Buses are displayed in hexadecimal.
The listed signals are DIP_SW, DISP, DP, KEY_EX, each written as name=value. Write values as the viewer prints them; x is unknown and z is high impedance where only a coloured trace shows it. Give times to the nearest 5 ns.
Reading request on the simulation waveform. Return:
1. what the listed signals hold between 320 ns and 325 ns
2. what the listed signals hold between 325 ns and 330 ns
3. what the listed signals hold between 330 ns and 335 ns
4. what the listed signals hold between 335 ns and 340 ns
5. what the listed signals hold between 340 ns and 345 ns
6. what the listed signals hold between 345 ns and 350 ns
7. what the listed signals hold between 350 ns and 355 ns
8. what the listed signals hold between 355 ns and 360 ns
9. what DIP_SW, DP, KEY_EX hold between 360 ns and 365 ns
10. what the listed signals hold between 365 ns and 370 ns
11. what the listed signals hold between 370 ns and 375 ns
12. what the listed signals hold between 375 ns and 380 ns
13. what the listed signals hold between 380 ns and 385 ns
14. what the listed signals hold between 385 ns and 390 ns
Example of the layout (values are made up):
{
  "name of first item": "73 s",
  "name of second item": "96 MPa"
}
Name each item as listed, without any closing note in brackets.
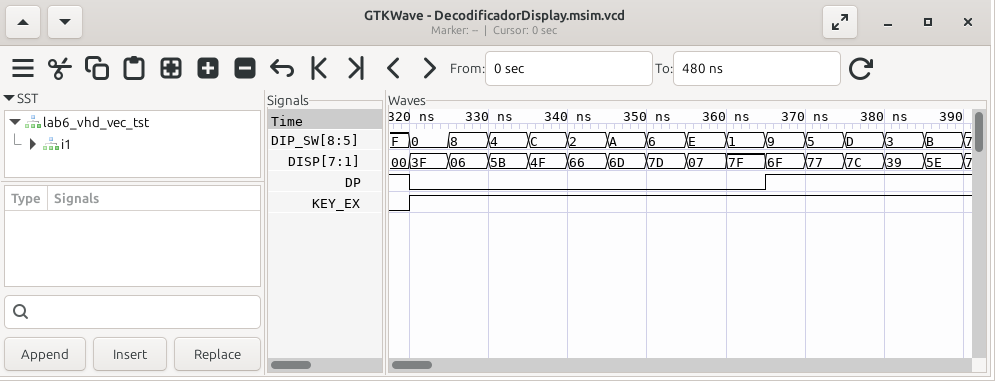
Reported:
{
  "what the listed signals hold between 320 ns and 325 ns": "DIP_SW=0, DISP=3F, DP=0, KEY_EX=1",
  "what the listed signals hold between 325 ns and 330 ns": "DIP_SW=8, DISP=06, DP=0, KEY_EX=1",
  "what the listed signals hold between 330 ns and 335 ns": "DIP_SW=4, DISP=5B, DP=0, KEY_EX=1",
  "what the listed signals hold between 335 ns and 340 ns": "DIP_SW=C, DISP=4F, DP=0, KEY_EX=1",
  "what the listed signals hold between 340 ns and 345 ns": "DIP_SW=2, DISP=66, DP=0, KEY_EX=1",
  "what the listed signals hold between 345 ns and 350 ns": "DIP_SW=A, DISP=6D, DP=0, KEY_EX=1",
  "what the listed signals hold between 350 ns and 355 ns": "DIP_SW=6, DISP=7D, DP=0, KEY_EX=1",
  "what the listed signals hold between 355 ns and 360 ns": "DIP_SW=E, DISP=07, DP=0, KEY_EX=1",
  "what DIP_SW, DP, KEY_EX hold between 360 ns and 365 ns": "DIP_SW=1, DP=0, KEY_EX=1",
  "what the listed signals hold between 365 ns and 370 ns": "DIP_SW=9, DISP=6F, DP=1, KEY_EX=1",
  "what the listed signals hold between 370 ns and 375 ns": "DIP_SW=5, DISP=77, DP=1, KEY_EX=1",
  "what the listed signals hold between 375 ns and 380 ns": "DIP_SW=D, DISP=7C, DP=1, KEY_EX=1",
  "what the listed signals hold between 380 ns and 385 ns": "DIP_SW=3, DISP=39, DP=1, KEY_EX=1",
  "what the listed signals hold between 385 ns and 390 ns": "DIP_SW=B, DISP=5E, DP=1, KEY_EX=1"
}
